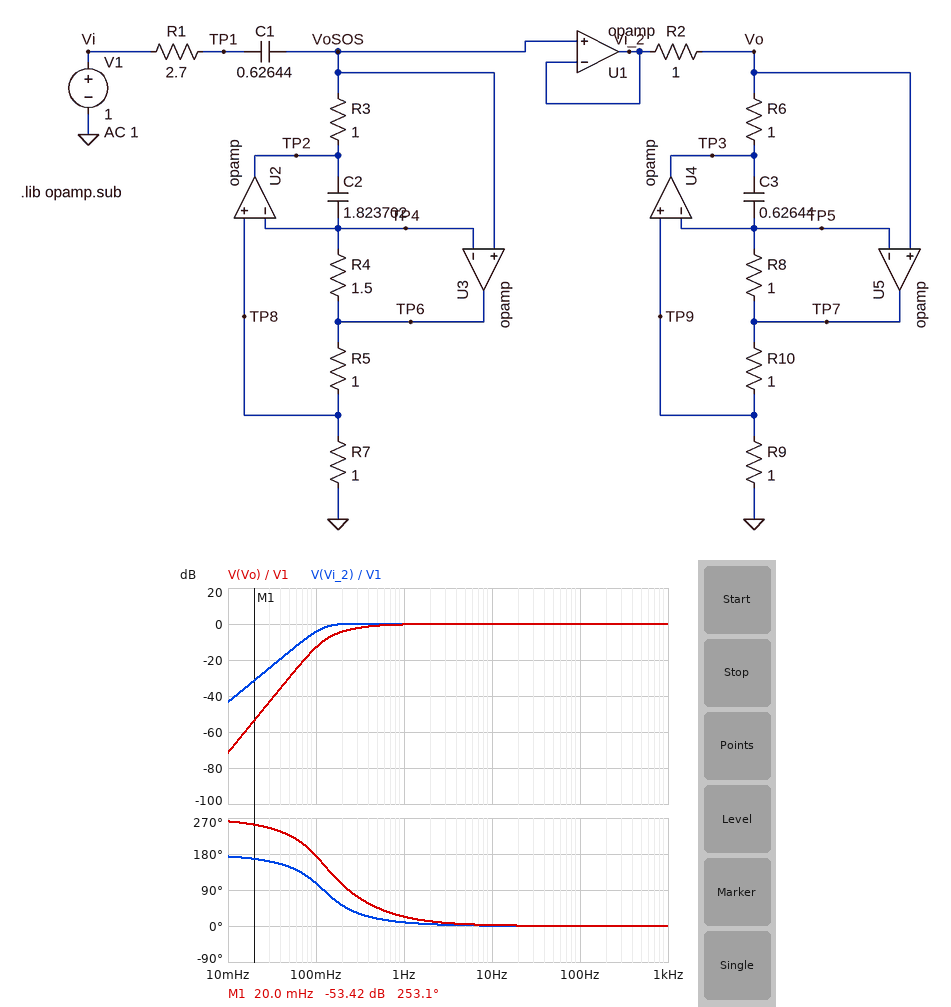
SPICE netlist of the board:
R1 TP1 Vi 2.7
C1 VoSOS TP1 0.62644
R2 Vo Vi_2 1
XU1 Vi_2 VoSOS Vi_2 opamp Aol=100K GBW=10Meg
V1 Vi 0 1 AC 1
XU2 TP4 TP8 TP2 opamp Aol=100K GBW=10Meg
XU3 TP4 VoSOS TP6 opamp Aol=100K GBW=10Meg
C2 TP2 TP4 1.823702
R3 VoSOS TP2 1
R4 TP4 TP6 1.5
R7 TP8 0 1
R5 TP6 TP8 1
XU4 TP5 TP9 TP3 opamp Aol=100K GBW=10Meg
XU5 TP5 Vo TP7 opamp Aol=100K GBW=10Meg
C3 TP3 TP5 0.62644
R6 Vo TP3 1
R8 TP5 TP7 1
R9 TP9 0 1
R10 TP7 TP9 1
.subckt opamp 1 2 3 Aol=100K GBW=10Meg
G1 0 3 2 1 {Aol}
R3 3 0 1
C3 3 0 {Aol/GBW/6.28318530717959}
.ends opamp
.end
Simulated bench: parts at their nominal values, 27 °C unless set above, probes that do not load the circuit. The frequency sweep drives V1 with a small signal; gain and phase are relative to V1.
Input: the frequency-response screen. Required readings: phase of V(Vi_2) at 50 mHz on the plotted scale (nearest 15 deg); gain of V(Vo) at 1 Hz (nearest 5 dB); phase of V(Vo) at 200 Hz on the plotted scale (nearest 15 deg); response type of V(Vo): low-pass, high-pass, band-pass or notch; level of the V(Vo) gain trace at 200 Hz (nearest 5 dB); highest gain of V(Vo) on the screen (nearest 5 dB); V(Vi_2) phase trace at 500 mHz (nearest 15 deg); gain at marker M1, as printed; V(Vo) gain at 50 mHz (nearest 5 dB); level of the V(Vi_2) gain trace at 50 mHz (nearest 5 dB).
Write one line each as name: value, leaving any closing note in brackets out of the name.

phase of V(Vi_2) at 50 mHz on the plotted scale: 150 deg
gain of V(Vo) at 1 Hz: 0 dB
phase of V(Vo) at 200 Hz on the plotted scale: 0 deg
response type of V(Vo): low-pass, high-pass, band-pass or notch: high-pass
level of the V(Vo) gain trace at 200 Hz: 0 dB
highest gain of V(Vo) on the screen: 0 dB
V(Vi_2) phase trace at 500 mHz: 15 deg
gain at marker M1, as printed: -53.42 dB
V(Vo) gain at 50 mHz: -30 dB
level of the V(Vi_2) gain trace at 50 mHz: -15 dB
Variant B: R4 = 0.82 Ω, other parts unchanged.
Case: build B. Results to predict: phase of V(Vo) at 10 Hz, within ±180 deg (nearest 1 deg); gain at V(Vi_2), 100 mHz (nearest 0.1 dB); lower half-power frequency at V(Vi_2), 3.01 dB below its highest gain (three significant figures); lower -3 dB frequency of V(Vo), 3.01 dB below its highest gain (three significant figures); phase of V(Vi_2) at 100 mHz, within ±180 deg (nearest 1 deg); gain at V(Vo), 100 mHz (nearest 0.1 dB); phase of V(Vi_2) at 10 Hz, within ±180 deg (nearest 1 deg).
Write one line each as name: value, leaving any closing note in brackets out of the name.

phase of V(Vo) at 10 Hz, within ±180 deg: 3 deg
gain at V(Vi_2), 100 mHz: -10.5 dB
lower half-power frequency at V(Vi_2), 3.01 dB below its highest gain: 212 mHz
lower -3 dB frequency of V(Vo), 3.01 dB below its highest gain: 344 mHz
phase of V(Vi_2) at 100 mHz, within ±180 deg: 121 deg
gain at V(Vo), 100 mHz: -19.2 dB
phase of V(Vi_2) at 10 Hz, within ±180 deg: 2 deg
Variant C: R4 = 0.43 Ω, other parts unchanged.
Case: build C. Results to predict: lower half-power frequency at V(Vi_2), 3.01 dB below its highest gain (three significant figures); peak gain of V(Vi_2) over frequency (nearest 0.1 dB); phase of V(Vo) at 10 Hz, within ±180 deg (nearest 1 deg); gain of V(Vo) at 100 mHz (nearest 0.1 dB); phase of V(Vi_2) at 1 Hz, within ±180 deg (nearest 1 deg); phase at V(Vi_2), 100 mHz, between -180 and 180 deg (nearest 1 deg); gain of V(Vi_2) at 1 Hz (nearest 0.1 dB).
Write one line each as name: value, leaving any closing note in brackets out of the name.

lower half-power frequency at V(Vi_2), 3.01 dB below its highest gain: 458 mHz
peak gain of V(Vi_2) over frequency: 0 dB
phase of V(Vo) at 10 Hz, within ±180 deg: 5 deg
gain of V(Vo) at 100 mHz: -25.5 dB
phase of V(Vi_2) at 1 Hz, within ±180 deg: 30 deg
phase at V(Vi_2), 100 mHz, between -180 and 180 deg: 127 deg
gain of V(Vi_2) at 1 Hz: -0.8 dB
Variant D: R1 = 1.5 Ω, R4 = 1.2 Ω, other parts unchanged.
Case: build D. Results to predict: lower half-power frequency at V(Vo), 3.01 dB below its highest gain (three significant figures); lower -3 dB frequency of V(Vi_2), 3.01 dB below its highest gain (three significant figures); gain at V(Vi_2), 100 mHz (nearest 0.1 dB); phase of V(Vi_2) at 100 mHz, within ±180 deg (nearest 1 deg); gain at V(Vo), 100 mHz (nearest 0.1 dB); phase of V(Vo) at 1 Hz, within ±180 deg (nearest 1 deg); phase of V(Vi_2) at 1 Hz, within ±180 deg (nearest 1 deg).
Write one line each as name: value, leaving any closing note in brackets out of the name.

lower half-power frequency at V(Vo), 3.01 dB below its highest gain: 156 mHz
lower -3 dB frequency of V(Vi_2), 3.01 dB below its highest gain: 114 mHz
gain at V(Vi_2), 100 mHz: -2.8 dB
phase of V(Vi_2) at 100 mHz, within ±180 deg: 128 deg
gain at V(Vo), 100 mHz: -11.5 dB
phase of V(Vo) at 1 Hz, within ±180 deg: 21 deg
phase of V(Vi_2) at 1 Hz, within ±180 deg: 6 deg
